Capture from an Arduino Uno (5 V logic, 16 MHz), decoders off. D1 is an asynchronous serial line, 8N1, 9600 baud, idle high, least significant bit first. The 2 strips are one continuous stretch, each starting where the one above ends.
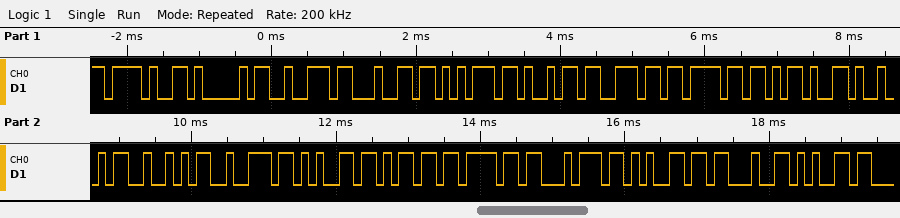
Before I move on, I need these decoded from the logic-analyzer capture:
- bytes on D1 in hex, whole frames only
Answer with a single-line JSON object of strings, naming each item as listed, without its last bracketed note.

{"bytes on D1 in hex, whole frames only": "0x2F 0x41 0x72 0x64 0x75 0x69 0x6E 0x6F 0x2D 0x49 0x52 0x72 0x65 0x6D 0x6F 0x74 0x65 0x23 0x65"}
